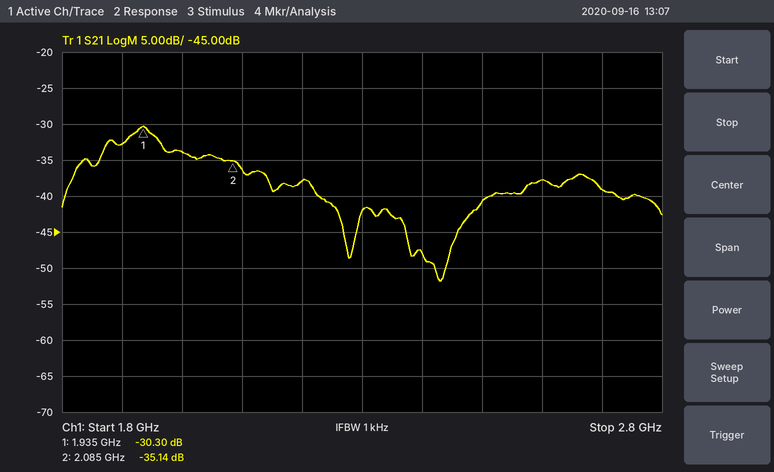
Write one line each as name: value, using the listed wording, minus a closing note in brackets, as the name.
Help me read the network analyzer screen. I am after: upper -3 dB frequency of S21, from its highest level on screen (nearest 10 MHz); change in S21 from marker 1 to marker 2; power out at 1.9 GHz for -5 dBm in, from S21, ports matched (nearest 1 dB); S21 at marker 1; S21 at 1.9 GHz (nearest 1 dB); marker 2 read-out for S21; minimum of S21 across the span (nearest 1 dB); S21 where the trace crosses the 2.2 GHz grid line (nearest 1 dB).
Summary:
upper -3 dB frequency of S21, from its highest level on screen: 1.97 GHz
change in S21 from marker 1 to marker 2: -4.84 dB
power out at 1.9 GHz for -5 dBm in, from S21, ports matched: -38 dBm
S21 at marker 1: -30.30 dB
S21 at 1.9 GHz: -33 dB
marker 2 read-out for S21: -35.14 dB
minimum of S21 across the span: -52 dB
S21 where the trace crosses the 2.2 GHz grid line: -38 dB
